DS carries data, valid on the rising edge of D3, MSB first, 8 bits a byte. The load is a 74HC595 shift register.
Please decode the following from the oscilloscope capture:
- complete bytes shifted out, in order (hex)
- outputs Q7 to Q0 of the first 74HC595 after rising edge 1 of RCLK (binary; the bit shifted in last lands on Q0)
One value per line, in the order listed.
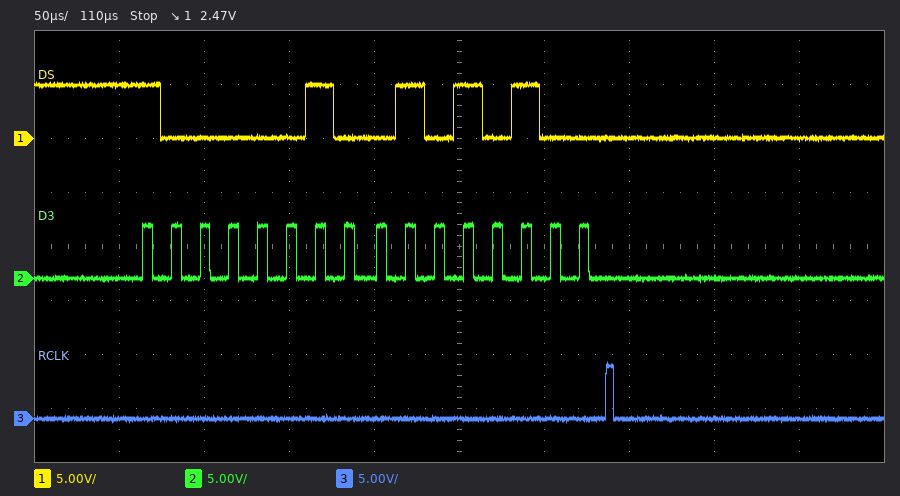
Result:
0x82 0x54
01010100
